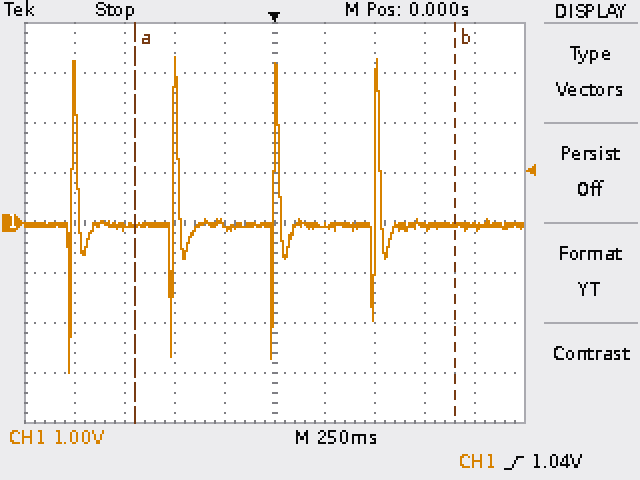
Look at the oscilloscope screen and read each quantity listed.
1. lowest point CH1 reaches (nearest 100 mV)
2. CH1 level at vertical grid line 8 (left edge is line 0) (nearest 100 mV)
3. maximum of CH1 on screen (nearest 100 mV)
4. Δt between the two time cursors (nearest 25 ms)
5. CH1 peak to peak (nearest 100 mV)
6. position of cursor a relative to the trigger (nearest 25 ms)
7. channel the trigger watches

-3.0 V
-100 mV
3.3 V
1.600 s
6.3 V
-700 ms
CH1
